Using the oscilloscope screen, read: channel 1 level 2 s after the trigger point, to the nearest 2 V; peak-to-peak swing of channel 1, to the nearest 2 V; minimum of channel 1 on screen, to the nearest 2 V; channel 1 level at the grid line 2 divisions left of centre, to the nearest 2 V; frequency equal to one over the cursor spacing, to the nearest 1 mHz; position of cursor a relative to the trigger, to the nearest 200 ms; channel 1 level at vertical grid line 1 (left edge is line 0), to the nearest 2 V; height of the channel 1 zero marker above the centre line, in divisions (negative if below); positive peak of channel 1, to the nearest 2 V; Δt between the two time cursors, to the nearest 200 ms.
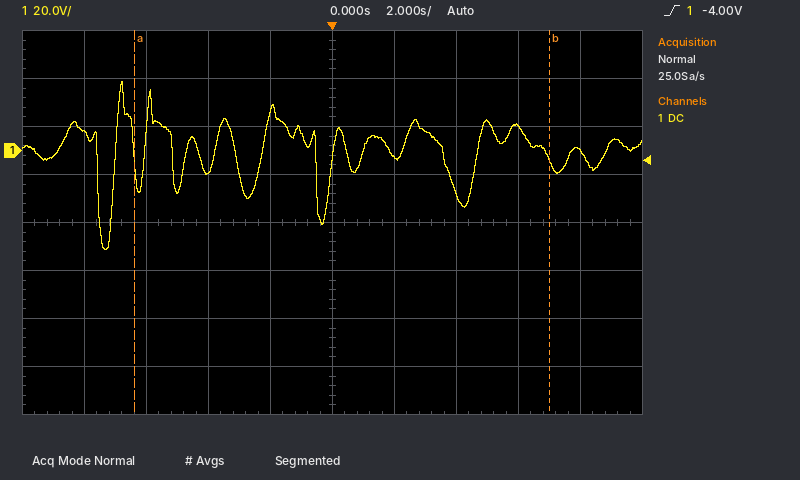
-2 V
70 V
-42 V
-8 V
75 mHz
-6.4 s
8 V
+1.5 div
28 V
13.4 s
